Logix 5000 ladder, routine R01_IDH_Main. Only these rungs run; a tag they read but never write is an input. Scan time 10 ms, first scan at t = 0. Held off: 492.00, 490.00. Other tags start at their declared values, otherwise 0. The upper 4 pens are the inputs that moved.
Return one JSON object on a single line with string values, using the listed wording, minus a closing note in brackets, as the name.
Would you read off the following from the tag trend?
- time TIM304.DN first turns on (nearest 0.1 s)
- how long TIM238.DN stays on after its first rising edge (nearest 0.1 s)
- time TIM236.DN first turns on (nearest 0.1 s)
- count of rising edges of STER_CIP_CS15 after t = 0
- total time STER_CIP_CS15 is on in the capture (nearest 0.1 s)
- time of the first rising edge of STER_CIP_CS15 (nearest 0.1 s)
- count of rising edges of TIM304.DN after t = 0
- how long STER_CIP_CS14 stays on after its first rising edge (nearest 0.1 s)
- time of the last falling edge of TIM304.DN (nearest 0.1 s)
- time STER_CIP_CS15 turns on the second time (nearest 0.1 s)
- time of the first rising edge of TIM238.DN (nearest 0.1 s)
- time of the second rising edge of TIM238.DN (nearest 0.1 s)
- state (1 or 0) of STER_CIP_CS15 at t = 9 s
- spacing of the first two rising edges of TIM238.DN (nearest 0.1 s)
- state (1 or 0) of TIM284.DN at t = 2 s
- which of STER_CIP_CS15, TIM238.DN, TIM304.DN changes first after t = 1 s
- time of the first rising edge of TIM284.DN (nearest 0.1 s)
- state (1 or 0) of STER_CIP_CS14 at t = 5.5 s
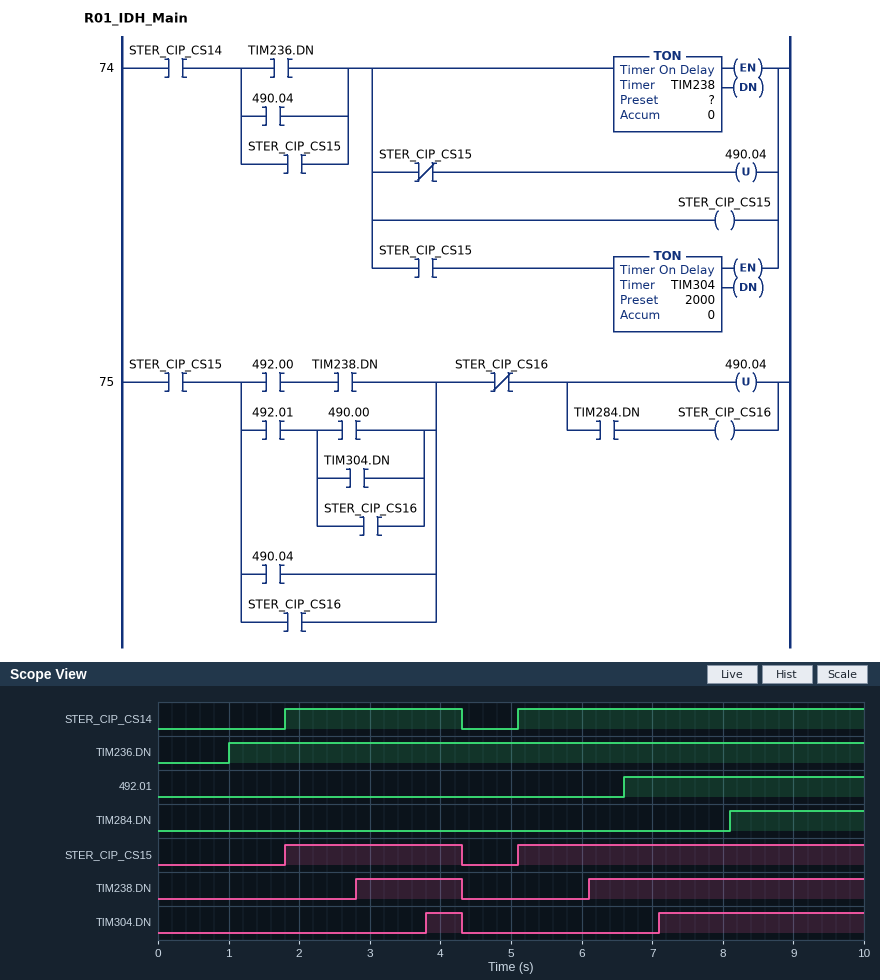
{"time TIM304.DN first turns on": "3.8 s", "how long TIM238.DN stays on after its first rising edge": "1.5 s", "time TIM236.DN first turns on": "1.0 s", "count of rising edges of STER_CIP_CS15 after t = 0": "2", "total time STER_CIP_CS15 is on in the capture": "7.4 s", "time of the first rising edge of STER_CIP_CS15": "1.8 s", "count of rising edges of TIM304.DN after t = 0": "2", "how long STER_CIP_CS14 stays on after its first rising edge": "2.5 s", "time of the last falling edge of TIM304.DN": "4.3 s", "time STER_CIP_CS15 turns on the second time": "5.1 s", "time of the first rising edge of TIM238.DN": "2.8 s", "time of the second rising edge of TIM238.DN": "6.1 s", "state (1 or 0) of STER_CIP_CS15 at t = 9 s": "1", "spacing of the first two rising edges of TIM238.DN": "3.3 s", "state (1 or 0) of TIM284.DN at t = 2 s": "0", "which of STER_CIP_CS15, TIM238.DN, TIM304.DN changes first after t = 1 s": "STER_CIP_CS15", "time of the first rising edge of TIM284.DN": "8.1 s", "state (1 or 0) of STER_CIP_CS14 at t = 5.5 s": "1"}
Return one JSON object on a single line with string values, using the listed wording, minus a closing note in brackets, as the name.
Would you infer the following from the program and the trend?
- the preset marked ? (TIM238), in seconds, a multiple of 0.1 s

{"the preset marked ? (TIM238), in seconds, a multiple of 0.1 s": "1.0 s"}
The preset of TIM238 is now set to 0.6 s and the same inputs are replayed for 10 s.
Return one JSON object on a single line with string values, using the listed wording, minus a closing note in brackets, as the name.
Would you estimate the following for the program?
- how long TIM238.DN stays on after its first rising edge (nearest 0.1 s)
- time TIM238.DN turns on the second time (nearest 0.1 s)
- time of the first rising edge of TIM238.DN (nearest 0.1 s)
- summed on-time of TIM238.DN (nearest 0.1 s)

{"how long TIM238.DN stays on after its first rising edge": "1.9 s", "time TIM238.DN turns on the second time": "5.7 s", "time of the first rising edge of TIM238.DN": "2.4 s", "summed on-time of TIM238.DN": "6.2 s"}
